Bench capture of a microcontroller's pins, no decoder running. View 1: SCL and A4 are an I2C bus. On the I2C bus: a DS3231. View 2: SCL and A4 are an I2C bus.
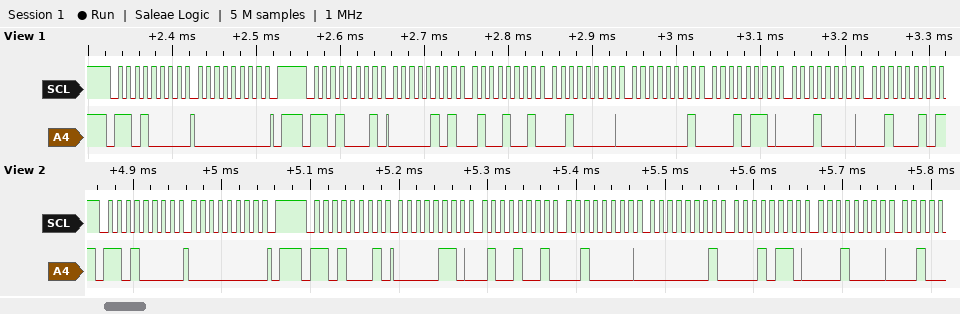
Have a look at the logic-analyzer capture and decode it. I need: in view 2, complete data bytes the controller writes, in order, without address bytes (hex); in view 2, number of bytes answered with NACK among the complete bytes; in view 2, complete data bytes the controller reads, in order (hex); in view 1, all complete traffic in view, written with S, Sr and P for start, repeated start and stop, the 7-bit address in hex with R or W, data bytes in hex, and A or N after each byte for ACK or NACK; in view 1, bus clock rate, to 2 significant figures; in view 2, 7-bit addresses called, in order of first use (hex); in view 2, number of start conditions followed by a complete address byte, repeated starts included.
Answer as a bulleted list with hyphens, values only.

- 00
- 0
- 06 49 20 01 16 10
- S 68W A 00 A P S 68R A 05 A 49 A 20 A 01 A 16 A 10 A 22 N
- 100 kHz
- 0x68
- 2
